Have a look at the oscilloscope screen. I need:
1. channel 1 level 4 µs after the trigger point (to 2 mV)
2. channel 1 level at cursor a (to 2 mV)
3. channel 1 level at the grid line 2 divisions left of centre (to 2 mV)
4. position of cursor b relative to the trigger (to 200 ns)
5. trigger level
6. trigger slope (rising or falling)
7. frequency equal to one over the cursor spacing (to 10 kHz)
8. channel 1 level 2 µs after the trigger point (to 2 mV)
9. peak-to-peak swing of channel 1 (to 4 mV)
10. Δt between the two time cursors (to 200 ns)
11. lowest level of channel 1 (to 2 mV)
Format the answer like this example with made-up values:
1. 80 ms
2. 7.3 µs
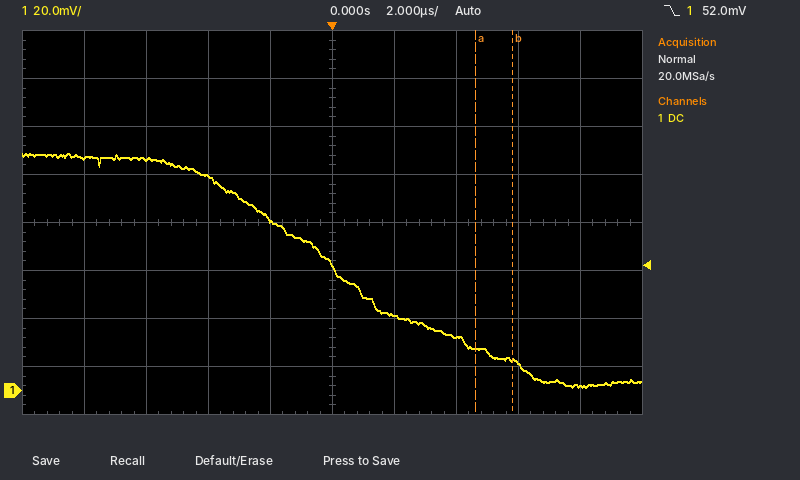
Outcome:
1. 22 mV
2. 18 mV
3. 90 mV
4. +5.8 µs
5. 52.0 mV
6. falling
7. 830 kHz
8. 32 mV
9. 96 mV
10. 1.2 µs
11. 2 mV
